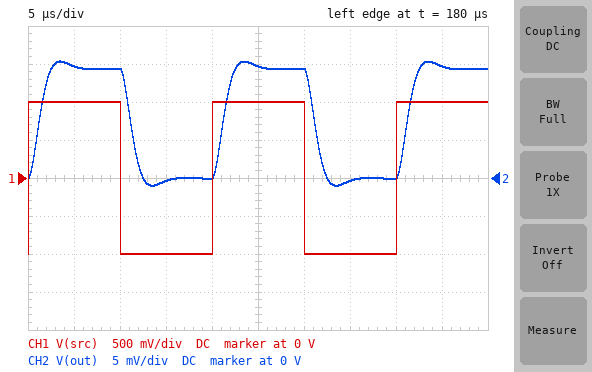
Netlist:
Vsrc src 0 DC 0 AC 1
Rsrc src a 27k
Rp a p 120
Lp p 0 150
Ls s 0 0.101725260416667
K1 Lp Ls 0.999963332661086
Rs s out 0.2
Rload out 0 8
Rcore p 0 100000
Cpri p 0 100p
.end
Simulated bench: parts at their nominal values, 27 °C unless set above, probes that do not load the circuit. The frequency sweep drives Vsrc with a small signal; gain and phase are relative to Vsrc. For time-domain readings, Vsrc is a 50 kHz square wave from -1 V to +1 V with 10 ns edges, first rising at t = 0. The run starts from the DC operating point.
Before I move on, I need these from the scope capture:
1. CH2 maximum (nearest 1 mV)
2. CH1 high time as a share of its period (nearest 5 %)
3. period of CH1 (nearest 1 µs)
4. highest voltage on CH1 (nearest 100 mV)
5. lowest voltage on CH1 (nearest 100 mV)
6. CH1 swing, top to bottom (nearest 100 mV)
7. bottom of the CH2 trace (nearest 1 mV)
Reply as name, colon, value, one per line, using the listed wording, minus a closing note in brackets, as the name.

CH2 maximum: 15 mV
CH1 high time as a share of its period: 50 %
period of CH1: 20 µs
highest voltage on CH1: 1.0 V
lowest voltage on CH1: -1.0 V
CH1 swing, top to bottom: 2.0 V
bottom of the CH2 trace: -1 mV
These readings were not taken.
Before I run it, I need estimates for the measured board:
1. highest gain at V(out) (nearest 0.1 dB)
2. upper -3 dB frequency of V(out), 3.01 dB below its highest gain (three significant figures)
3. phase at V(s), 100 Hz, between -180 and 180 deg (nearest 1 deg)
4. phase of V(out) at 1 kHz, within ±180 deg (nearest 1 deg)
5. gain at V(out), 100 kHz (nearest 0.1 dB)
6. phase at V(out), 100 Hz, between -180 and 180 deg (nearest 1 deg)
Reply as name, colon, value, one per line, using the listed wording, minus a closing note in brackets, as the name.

highest gain at V(out): -42.7 dB
upper -3 dB frequency of V(out), 3.01 dB below its highest gain: 202 kHz
phase at V(s), 100 Hz, between -180 and 180 deg: 5 deg
phase of V(out) at 1 kHz, within ±180 deg: 0 deg
gain at V(out), 100 kHz: -42.8 dB
phase at V(out), 100 Hz, between -180 and 180 deg: 5 deg
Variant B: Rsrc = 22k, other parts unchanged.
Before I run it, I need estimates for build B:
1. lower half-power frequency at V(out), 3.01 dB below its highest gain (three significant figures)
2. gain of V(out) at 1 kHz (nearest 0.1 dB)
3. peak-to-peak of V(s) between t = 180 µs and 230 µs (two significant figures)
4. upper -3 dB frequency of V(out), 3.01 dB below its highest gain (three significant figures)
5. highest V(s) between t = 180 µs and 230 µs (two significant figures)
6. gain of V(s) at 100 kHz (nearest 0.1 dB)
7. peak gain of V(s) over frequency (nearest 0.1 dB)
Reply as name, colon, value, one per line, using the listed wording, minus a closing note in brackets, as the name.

lower half-power frequency at V(out), 3.01 dB below its highest gain: 7.77 Hz
gain of V(out) at 1 kHz: -41.6 dB
peak-to-peak of V(s) between t = 180 µs and 230 µs: 19 mV
upper -3 dB frequency of V(out), 3.01 dB below its highest gain: 205 kHz
highest V(s) between t = 180 µs and 230 µs: 18 mV
gain of V(s) at 100 kHz: -41.4 dB
peak gain of V(s) over frequency: -41.3 dB
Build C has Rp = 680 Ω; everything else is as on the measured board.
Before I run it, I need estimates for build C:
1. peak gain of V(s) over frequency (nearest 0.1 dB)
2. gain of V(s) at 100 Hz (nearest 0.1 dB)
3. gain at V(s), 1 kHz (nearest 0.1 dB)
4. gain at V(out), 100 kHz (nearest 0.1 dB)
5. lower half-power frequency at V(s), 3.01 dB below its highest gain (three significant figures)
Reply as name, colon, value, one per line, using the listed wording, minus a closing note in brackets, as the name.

peak gain of V(s) over frequency: -42.6 dB
gain of V(s) at 100 Hz: -42.8 dB
gain at V(s), 1 kHz: -42.7 dB
gain at V(out), 100 kHz: -42.9 dB
lower half-power frequency at V(s), 3.01 dB below its highest gain: 8.40 Hz
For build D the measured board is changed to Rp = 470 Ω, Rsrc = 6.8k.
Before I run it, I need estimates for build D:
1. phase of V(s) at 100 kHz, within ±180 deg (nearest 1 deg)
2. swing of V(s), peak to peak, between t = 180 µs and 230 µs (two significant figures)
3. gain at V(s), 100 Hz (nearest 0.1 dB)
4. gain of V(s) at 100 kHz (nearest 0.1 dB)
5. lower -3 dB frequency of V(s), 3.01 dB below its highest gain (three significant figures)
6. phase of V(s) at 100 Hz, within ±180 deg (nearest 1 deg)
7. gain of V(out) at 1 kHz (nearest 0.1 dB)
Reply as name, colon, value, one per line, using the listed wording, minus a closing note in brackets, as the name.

phase of V(s) at 100 kHz, within ±180 deg: -37 deg
swing of V(s), peak to peak, between t = 180 µs and 230 µs: 32 mV
gain at V(s), 100 Hz: -36.2 dB
gain of V(s) at 100 kHz: -36.7 dB
lower -3 dB frequency of V(s), 3.01 dB below its highest gain: 4.61 Hz
phase of V(s) at 100 Hz, within ±180 deg: 3 deg
gain of V(out) at 1 kHz: -36.4 dB
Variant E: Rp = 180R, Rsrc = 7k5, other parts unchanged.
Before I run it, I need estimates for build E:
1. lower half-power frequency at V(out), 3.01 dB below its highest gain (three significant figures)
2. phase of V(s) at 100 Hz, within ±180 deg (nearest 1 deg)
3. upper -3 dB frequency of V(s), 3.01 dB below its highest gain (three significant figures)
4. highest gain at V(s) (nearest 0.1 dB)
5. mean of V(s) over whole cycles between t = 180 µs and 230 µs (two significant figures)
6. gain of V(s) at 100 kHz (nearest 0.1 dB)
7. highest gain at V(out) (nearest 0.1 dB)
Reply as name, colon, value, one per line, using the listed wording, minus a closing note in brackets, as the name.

lower half-power frequency at V(out), 3.01 dB below its highest gain: 4.76 Hz
phase of V(s) at 100 Hz, within ±180 deg: 3 deg
upper -3 dB frequency of V(s), 3.01 dB below its highest gain: 217 kHz
highest gain at V(s): -36.4 dB
mean of V(s) over whole cycles between t = 180 µs and 230 µs: 15 mV
gain of V(s) at 100 kHz: -36.8 dB
highest gain at V(out): -36.6 dB
